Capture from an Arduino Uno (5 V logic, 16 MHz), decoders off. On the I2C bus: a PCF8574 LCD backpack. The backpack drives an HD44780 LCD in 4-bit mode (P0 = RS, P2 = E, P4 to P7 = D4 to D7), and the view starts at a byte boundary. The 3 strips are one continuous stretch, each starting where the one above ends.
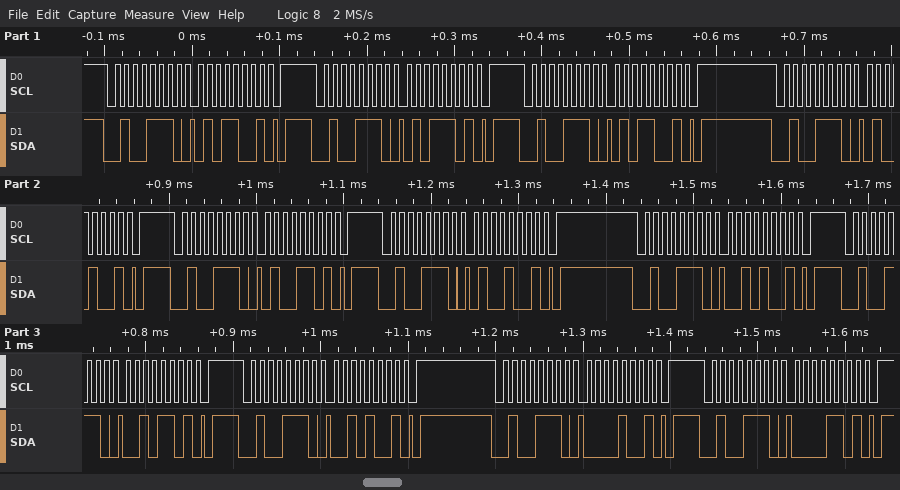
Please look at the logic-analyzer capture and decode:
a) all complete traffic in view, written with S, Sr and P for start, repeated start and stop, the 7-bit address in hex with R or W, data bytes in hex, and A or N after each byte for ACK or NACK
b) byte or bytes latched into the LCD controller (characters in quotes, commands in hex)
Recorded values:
S 27W A 59 A P S 27W A 5D A P S 27W A 59 A P S 27W A 49 A P S 27W A 4D A P S 27W A 49 A P S 27W A 29 A P S 27W A 2D A P S 27W A 29 A P S 27W A 09 A P S 27W A 0D A P
'T'
